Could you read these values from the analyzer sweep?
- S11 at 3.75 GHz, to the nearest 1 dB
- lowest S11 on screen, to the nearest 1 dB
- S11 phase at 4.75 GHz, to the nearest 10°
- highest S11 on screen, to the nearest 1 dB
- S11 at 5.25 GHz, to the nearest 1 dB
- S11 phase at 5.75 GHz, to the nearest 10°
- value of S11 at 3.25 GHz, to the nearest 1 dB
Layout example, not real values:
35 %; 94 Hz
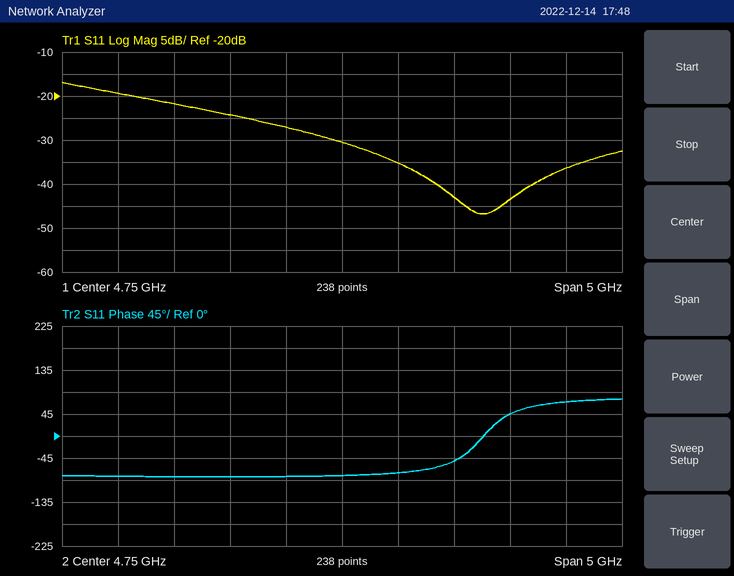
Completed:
-24 dB; -47 dB; -80°; -17 dB; -35 dB; -50°; -22 dB
